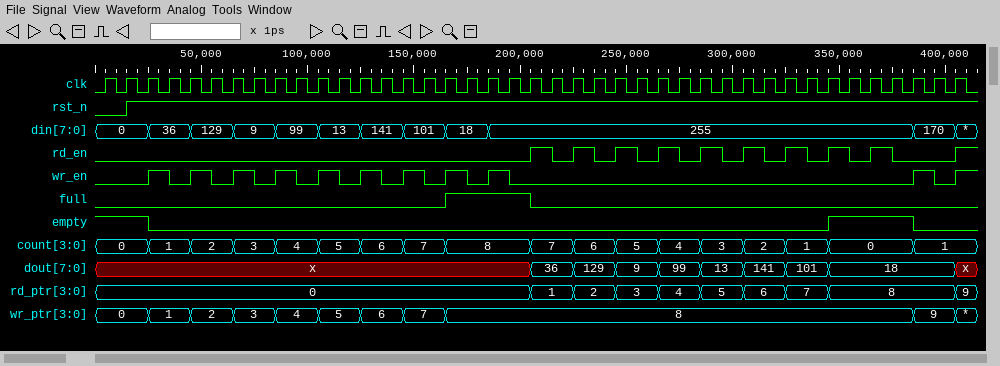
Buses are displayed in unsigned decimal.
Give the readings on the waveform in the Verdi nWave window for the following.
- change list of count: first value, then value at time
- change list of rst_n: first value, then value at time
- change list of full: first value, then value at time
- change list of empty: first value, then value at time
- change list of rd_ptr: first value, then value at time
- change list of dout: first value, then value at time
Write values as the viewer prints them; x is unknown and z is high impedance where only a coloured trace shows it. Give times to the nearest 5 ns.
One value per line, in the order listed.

0, 1 at 25 ns, 2 at 45 ns, 3 at 65 ns, 4 at 85 ns, 5 at 105 ns, 6 at 125 ns, 7 at 145 ns, 8 at 165 ns, 7 at 205 ns, 6 at 225 ns, 5 at 245 ns, 4 at 265 ns, 3 at 285 ns, 2 at 305 ns, 1 at 325 ns, 0 at 345 ns, 1 at 385 ns
0, 1 at 15 ns
0, 1 at 165 ns, 0 at 205 ns
1, 0 at 25 ns, 1 at 345 ns, 0 at 385 ns
0, 1 at 205 ns, 2 at 225 ns, 3 at 245 ns, 4 at 265 ns, 5 at 285 ns, 6 at 305 ns, 7 at 325 ns, 8 at 345 ns, 9 at 405 ns
x, 36 at 205 ns, 129 at 225 ns, 9 at 245 ns, 99 at 265 ns, 13 at 285 ns, 141 at 305 ns, 101 at 325 ns, 18 at 345 ns, x at 405 ns
